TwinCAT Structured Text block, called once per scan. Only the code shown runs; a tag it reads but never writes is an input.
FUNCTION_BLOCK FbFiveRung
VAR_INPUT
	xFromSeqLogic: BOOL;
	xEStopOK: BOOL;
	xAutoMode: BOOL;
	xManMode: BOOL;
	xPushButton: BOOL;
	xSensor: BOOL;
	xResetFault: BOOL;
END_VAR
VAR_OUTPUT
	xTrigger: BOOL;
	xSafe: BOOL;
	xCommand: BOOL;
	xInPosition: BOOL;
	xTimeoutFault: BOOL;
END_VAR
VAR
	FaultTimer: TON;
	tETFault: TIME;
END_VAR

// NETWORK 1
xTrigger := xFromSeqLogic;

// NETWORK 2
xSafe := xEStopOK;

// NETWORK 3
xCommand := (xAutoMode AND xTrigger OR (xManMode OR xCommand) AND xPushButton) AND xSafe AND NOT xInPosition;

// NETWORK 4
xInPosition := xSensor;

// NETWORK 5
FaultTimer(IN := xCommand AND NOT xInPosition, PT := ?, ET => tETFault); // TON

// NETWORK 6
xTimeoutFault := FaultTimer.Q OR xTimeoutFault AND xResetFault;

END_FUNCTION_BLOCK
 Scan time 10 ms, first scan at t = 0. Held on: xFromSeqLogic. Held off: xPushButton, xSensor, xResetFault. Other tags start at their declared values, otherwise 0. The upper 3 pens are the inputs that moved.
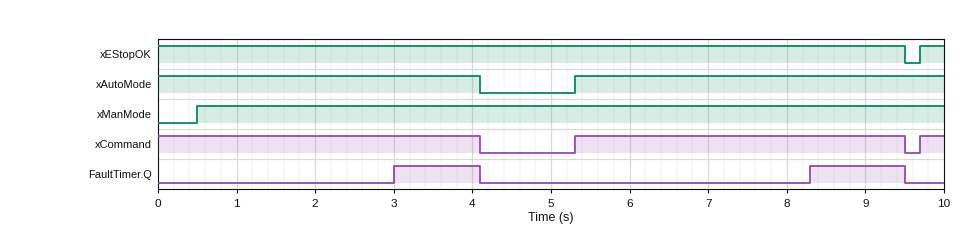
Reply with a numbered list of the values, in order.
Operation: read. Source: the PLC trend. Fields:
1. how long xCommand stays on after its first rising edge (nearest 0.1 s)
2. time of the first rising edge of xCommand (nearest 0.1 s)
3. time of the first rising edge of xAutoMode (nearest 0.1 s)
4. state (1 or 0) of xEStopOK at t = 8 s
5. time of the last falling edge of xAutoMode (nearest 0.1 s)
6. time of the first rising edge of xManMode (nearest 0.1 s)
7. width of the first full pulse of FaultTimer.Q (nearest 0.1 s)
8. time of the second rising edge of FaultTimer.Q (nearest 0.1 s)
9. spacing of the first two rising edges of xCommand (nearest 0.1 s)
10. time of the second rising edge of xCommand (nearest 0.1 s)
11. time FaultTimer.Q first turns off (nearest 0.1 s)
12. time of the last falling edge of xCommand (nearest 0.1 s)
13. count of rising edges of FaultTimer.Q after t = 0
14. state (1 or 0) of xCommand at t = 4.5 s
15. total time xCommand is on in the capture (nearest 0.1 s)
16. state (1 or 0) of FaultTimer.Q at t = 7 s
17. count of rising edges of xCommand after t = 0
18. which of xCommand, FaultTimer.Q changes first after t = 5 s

1. 4.2 s
2. 5.3 s
3. 5.3 s
4. 1
5. 4.1 s
6. 0.5 s
7. 1.1 s
8. 8.3 s
9. 4.4 s
10. 9.7 s
11. 4.1 s
12. 9.5 s
13. 2
14. 0
15. 8.6 s
16. 0
17. 2
18. xCommand
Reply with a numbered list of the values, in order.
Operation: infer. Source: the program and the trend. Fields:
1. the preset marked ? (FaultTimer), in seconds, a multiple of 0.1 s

1. 3.0 s
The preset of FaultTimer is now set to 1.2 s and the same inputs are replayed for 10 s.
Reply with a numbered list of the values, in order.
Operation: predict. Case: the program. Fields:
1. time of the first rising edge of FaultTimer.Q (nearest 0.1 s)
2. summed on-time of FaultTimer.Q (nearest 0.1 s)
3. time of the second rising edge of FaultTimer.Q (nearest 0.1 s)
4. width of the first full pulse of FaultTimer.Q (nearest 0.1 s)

1. 1.2 s
2. 5.9 s
3. 6.5 s
4. 2.9 s
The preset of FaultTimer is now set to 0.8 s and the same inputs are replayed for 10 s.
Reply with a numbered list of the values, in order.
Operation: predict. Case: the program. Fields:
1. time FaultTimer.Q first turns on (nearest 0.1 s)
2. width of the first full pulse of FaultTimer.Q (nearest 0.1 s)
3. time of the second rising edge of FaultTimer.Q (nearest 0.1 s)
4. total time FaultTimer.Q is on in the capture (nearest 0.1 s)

1. 0.8 s
2. 3.3 s
3. 6.1 s
4. 6.7 s
